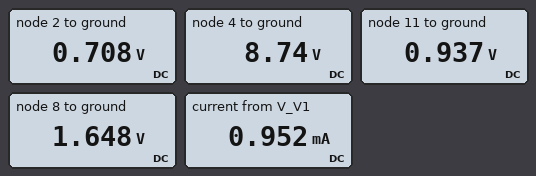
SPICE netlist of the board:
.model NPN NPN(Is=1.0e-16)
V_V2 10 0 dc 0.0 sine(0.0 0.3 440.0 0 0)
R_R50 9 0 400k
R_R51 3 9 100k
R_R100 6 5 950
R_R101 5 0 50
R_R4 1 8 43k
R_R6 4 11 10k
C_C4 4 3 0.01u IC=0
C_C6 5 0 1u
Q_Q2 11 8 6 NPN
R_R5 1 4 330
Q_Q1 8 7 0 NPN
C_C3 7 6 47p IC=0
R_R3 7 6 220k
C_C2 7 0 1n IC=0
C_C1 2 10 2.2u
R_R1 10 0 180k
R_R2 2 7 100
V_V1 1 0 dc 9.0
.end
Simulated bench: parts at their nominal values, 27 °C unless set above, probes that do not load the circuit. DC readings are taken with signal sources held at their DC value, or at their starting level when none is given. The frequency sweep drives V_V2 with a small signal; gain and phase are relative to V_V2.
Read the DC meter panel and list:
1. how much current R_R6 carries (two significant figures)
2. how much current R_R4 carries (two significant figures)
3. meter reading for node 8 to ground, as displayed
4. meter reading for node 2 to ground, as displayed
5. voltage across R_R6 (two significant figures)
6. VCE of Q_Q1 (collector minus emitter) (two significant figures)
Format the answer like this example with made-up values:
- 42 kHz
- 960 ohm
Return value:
- 780 µA
- 170 µA
- 1.648 V
- 0.708 V
- 7.8 V
- 1.6 V
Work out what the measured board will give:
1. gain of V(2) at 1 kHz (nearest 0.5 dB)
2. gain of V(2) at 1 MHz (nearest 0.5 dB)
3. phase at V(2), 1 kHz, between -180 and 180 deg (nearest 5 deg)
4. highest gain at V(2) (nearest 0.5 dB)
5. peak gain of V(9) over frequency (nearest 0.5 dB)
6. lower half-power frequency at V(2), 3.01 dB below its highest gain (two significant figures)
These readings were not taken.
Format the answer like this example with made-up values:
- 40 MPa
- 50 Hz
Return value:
- 0 dB
- 0 dB
- 0 deg
- 0 dB
- -26.0 dB
- 3.3 Hz
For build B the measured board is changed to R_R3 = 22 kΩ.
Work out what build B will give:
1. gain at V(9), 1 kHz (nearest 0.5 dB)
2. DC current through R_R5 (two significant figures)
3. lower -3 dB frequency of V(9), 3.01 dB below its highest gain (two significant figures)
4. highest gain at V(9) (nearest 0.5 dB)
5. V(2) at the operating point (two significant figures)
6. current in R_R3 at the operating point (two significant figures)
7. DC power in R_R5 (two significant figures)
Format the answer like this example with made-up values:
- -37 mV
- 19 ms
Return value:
- 28.5 dB
- 760 µA
- 360 Hz
- 29.0 dB
- 730 mV
- 1.7 µA
- 190 µW
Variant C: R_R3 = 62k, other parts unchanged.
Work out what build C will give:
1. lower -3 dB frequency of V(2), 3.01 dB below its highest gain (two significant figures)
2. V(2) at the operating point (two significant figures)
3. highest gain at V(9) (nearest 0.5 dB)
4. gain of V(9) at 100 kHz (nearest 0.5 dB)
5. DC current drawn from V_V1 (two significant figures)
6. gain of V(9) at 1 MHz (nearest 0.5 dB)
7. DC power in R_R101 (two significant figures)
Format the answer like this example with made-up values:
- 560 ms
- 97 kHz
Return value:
- 11 Hz
- 720 mV
- -27.5 dB
- -33.5 dB
- 960 µA
- -29.0 dB
- 33 µW
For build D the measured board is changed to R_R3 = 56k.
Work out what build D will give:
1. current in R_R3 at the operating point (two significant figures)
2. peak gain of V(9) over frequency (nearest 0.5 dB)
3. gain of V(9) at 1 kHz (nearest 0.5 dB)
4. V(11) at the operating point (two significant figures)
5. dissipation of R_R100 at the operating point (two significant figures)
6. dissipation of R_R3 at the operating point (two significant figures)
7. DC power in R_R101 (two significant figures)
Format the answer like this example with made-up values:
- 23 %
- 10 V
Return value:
- 1.5 µA
- -24.0 dB
- -25.0 dB
- 910 mV
- 620 µW
- 120 nW
- 33 µW
